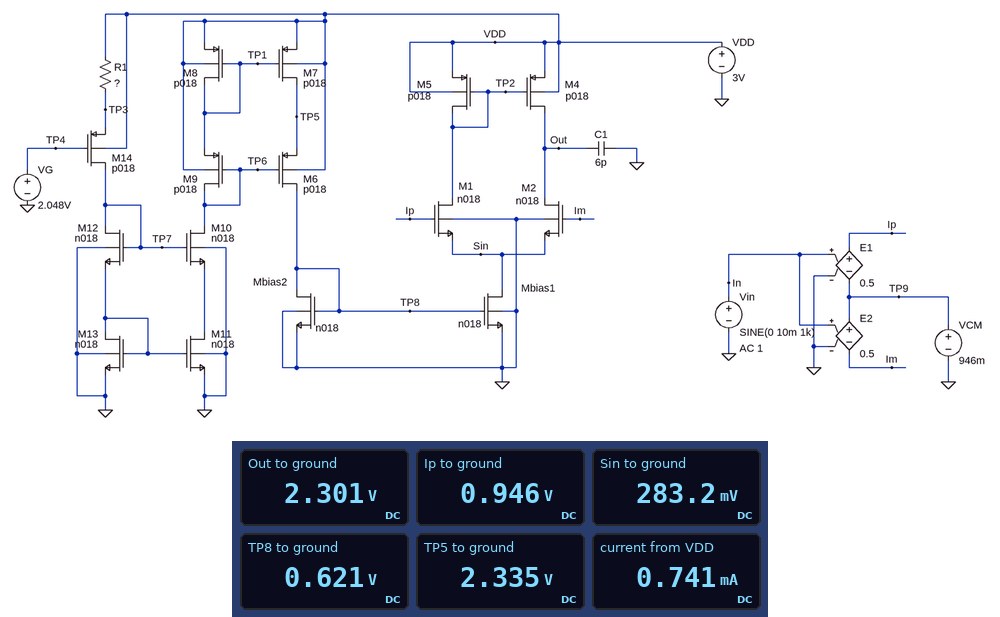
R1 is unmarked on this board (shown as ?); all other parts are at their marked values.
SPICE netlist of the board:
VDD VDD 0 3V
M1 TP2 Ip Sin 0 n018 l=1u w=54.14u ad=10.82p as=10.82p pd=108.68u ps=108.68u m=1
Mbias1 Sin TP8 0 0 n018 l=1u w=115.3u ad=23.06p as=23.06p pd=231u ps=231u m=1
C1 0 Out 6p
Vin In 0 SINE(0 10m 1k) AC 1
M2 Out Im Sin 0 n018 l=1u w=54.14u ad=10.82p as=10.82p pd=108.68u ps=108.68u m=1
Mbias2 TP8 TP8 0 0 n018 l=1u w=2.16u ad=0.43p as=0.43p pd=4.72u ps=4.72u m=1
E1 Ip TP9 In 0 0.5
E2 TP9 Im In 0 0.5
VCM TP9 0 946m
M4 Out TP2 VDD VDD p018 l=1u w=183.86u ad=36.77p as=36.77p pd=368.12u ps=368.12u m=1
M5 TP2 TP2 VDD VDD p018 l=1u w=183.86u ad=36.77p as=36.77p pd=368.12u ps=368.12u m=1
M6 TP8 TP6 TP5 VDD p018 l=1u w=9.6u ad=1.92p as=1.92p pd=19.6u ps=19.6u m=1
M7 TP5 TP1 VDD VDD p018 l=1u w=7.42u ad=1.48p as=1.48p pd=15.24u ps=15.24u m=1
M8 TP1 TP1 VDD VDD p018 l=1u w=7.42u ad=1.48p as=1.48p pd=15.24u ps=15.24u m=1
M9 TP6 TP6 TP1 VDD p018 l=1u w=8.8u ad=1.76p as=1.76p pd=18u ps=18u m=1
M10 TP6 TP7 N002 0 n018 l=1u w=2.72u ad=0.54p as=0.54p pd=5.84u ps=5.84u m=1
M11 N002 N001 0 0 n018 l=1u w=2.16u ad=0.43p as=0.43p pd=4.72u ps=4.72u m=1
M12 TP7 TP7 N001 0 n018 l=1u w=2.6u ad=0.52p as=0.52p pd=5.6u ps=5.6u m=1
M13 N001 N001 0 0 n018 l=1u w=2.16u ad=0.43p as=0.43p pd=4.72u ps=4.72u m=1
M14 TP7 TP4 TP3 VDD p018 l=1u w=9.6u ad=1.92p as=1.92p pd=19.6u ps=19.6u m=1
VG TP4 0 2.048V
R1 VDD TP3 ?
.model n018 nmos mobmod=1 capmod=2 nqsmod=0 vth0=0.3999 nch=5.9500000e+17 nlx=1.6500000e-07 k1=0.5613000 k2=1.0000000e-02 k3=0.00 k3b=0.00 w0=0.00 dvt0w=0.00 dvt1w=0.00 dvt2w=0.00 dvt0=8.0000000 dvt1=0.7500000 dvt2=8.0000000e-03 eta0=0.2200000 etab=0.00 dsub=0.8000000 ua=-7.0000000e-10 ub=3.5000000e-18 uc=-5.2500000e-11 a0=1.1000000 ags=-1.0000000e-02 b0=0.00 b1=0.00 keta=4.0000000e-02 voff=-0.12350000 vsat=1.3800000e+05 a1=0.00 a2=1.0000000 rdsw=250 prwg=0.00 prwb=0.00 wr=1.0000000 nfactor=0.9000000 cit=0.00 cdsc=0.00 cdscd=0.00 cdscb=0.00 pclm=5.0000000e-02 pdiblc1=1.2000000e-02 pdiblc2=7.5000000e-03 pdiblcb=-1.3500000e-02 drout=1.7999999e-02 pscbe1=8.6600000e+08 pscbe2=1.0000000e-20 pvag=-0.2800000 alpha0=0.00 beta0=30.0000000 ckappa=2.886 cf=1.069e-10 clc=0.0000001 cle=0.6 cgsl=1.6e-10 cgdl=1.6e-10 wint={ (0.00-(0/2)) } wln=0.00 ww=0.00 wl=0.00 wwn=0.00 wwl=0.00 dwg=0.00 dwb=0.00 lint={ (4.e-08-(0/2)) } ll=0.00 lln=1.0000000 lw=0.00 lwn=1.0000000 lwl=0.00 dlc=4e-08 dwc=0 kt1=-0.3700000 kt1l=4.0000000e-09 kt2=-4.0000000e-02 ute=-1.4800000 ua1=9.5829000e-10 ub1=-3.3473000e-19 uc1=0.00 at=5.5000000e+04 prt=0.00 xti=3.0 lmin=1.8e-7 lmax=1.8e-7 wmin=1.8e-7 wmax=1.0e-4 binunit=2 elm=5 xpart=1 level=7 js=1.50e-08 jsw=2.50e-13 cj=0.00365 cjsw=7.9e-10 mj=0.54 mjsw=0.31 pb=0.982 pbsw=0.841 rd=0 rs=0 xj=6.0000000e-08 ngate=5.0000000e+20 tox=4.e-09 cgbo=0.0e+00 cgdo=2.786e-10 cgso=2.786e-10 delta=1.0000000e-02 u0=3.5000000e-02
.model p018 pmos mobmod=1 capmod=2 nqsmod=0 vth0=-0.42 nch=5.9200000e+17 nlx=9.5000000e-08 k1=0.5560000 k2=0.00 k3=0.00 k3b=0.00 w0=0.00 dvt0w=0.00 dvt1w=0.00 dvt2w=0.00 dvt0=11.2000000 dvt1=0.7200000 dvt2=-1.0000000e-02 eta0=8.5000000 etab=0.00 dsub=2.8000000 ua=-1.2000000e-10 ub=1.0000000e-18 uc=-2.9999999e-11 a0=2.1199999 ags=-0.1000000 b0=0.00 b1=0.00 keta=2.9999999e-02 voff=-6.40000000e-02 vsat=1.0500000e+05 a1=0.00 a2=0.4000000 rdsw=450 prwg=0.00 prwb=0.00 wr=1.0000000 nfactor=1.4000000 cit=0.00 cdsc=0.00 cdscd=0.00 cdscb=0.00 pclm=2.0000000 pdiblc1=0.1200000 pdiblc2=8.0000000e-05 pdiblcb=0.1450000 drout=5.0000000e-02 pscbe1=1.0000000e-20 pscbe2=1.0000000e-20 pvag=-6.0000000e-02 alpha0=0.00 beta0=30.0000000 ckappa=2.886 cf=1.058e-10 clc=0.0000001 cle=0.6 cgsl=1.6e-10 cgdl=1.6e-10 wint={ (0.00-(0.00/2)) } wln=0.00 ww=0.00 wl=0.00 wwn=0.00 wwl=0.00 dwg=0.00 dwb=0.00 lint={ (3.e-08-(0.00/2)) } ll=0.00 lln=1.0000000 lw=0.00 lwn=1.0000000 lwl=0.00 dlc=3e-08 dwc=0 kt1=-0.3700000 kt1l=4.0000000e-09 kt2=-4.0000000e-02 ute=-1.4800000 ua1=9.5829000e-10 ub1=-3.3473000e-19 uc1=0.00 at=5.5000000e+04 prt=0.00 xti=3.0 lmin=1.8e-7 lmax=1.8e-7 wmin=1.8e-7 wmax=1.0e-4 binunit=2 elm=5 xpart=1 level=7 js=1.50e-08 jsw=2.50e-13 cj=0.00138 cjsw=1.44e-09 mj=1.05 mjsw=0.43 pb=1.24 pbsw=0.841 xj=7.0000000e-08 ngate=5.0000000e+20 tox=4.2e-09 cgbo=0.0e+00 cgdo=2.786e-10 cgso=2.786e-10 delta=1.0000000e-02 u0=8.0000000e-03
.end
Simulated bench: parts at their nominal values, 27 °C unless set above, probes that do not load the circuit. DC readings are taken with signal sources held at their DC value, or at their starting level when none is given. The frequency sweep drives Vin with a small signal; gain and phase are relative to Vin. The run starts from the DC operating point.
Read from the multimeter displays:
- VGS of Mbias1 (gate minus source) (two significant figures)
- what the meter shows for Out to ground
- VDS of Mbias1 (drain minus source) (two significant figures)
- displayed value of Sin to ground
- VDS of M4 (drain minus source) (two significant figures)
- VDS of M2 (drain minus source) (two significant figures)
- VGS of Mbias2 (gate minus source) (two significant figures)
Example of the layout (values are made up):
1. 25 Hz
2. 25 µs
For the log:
1. 620 mV
2. 2.301 V
3. 280 mV
4. 283.2 mV
5. -700 mV
6. 2.0 V
7. 620 mV
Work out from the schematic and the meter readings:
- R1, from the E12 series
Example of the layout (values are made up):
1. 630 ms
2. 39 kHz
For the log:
1. 33 kΩ
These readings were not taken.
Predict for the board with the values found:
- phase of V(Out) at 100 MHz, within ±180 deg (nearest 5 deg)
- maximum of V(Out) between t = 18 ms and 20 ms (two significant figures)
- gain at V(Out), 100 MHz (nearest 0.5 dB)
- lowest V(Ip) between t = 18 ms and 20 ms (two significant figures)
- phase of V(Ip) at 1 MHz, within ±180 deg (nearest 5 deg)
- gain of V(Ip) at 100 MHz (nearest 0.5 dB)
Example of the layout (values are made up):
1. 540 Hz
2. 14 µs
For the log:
1. -110 deg
2. 2.6 V
3. -7.0 dB
4. 940 mV
5. 0 deg
6. -6.0 dB
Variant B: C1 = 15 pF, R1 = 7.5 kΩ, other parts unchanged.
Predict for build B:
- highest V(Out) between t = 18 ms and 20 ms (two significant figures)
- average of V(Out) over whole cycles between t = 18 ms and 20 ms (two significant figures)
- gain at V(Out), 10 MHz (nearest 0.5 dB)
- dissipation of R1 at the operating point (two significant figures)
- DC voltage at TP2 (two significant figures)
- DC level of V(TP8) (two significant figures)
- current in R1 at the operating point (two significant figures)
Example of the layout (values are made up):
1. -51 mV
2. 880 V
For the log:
1. 2.4 V
2. 2.1 V
3. 9.0 dB
4. 3.7 µW
5. 2.2 V
6. 770 mV
7. 22 µA
